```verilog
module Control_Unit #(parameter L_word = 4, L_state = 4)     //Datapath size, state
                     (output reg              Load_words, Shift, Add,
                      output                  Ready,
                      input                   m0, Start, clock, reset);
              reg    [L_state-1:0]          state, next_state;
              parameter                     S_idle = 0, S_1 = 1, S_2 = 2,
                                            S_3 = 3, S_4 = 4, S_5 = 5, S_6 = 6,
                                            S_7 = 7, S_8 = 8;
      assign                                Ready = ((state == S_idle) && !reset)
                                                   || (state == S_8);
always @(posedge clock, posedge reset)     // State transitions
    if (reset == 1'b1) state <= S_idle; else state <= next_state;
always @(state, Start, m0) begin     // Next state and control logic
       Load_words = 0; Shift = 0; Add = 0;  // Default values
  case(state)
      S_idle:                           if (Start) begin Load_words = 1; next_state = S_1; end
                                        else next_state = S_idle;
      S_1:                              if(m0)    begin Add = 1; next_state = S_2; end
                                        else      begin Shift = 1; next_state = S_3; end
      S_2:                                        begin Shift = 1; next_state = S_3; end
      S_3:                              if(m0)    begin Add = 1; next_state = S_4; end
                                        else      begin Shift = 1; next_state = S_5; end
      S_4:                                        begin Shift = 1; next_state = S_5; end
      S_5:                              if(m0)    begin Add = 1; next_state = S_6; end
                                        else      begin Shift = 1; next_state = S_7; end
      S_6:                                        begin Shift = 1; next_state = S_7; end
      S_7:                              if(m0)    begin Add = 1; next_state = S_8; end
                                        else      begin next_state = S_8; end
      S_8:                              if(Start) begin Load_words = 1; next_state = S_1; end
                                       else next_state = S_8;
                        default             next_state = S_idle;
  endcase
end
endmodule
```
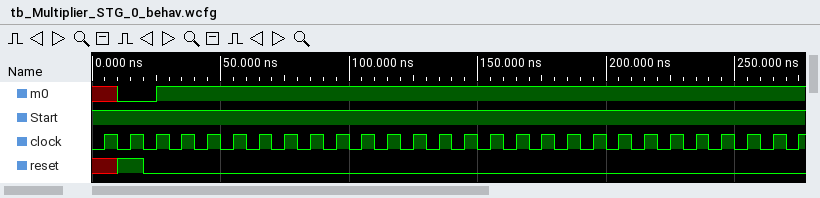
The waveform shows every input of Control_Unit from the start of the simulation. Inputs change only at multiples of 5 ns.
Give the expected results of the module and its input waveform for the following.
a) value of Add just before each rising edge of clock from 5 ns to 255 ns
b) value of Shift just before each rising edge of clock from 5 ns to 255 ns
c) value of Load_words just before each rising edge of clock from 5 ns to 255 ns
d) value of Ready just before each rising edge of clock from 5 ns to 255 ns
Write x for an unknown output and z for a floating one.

0 0 0 1 0 1 0 1 0 1 0 1 0 1 0 1 0 1 0 1 0 1 0 1 0 1
0 0 0 0 1 0 1 0 1 0 0 0 1 0 1 0 1 0 0 0 1 0 1 0 1 0
0 1 1 0 0 0 0 0 0 0 1 0 0 0 0 0 0 0 1 0 0 0 0 0 0 0
x 0 1 0 0 0 0 0 0 0 1 0 0 0 0 0 0 0 1 0 0 0 0 0 0 0
